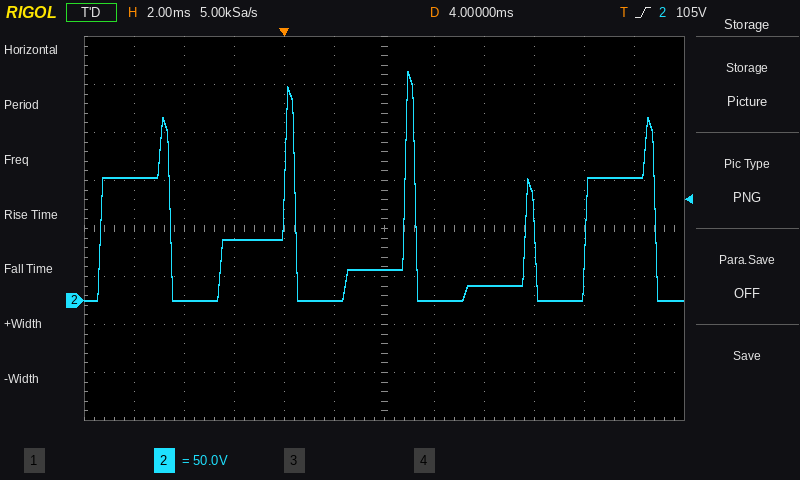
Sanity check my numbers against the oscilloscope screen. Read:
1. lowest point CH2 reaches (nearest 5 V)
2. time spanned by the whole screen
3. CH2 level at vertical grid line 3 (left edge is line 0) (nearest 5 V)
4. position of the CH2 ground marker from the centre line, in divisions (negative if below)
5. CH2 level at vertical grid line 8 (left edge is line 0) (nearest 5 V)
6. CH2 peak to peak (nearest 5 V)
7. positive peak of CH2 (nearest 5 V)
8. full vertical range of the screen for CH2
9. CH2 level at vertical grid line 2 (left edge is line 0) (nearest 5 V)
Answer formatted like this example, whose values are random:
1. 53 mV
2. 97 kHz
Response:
1. 0 V
2. 24 ms
3. 65 V
4. -1.5 div
5. 15 V
6. 240 V
7. 240 V
8. 400 V
9. 0 V
